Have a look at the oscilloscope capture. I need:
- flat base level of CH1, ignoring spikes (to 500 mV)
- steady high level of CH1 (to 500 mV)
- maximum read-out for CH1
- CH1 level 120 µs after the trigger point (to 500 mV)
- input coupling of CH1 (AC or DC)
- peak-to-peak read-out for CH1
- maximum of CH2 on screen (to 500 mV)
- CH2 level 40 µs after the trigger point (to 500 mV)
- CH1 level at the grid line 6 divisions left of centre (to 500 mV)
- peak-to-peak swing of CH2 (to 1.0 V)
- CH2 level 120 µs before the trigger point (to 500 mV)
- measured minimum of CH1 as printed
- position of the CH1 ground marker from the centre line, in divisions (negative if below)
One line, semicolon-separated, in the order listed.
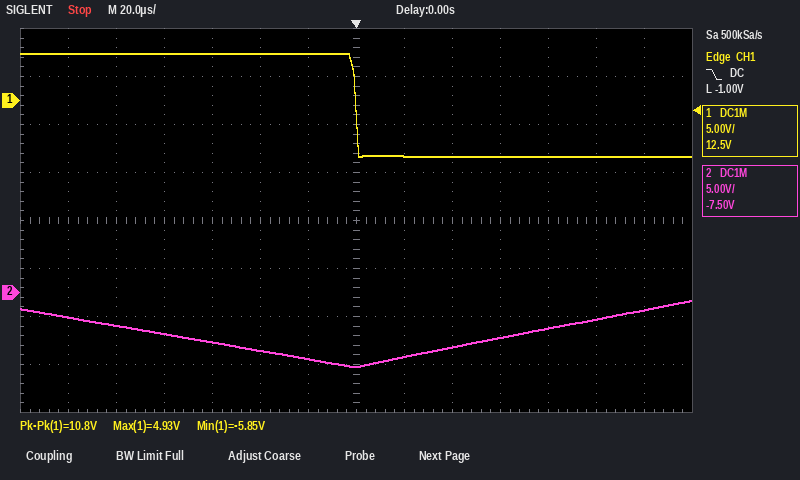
-6.0 V; 5.0 V; 4.93 V; -6.0 V; DC; 10.8 V; -1.0 V; -5.5 V; 5.0 V; 7.0 V; -2.5 V; -5.85 V; +2.5 div
